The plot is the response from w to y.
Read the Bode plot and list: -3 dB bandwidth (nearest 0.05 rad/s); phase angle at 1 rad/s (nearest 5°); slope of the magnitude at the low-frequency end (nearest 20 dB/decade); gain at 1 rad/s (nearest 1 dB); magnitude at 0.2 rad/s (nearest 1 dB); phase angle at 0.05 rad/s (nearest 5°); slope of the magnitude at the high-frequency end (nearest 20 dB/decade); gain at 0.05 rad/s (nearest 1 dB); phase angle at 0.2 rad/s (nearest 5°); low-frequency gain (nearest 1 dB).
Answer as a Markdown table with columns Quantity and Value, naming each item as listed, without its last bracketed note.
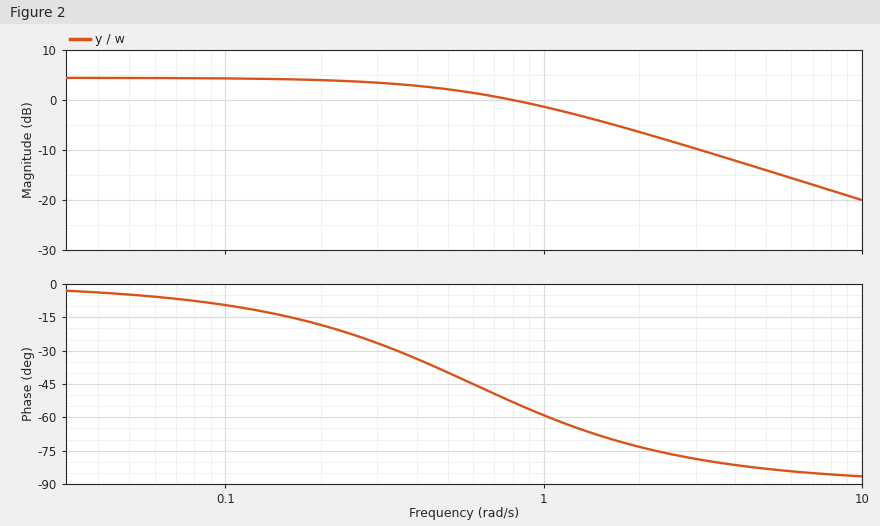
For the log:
| Quantity | Value |
|---|---|
| -3 dB bandwidth | 0.60 rad/s |
| phase angle at 1 rad/s | -60° |
| slope of the magnitude at the low-frequency end | 0 dB/decade |
| gain at 1 rad/s | -1 dB |
| magnitude at 0.2 rad/s | 4 dB |
| phase angle at 0.05 rad/s | -5° |
| slope of the magnitude at the high-frequency end | -20 dB/decade |
| gain at 0.05 rad/s | 4 dB |
| phase angle at 0.2 rad/s | -20° |
| low-frequency gain | 4 dB |
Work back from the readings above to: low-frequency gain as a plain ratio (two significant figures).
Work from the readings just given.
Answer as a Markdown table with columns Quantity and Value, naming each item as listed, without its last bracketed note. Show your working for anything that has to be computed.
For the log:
| Quantity | Value |
|---|---|
| low-frequency gain as a plain ratio | 10^(4 / 20) = 1.6 |
